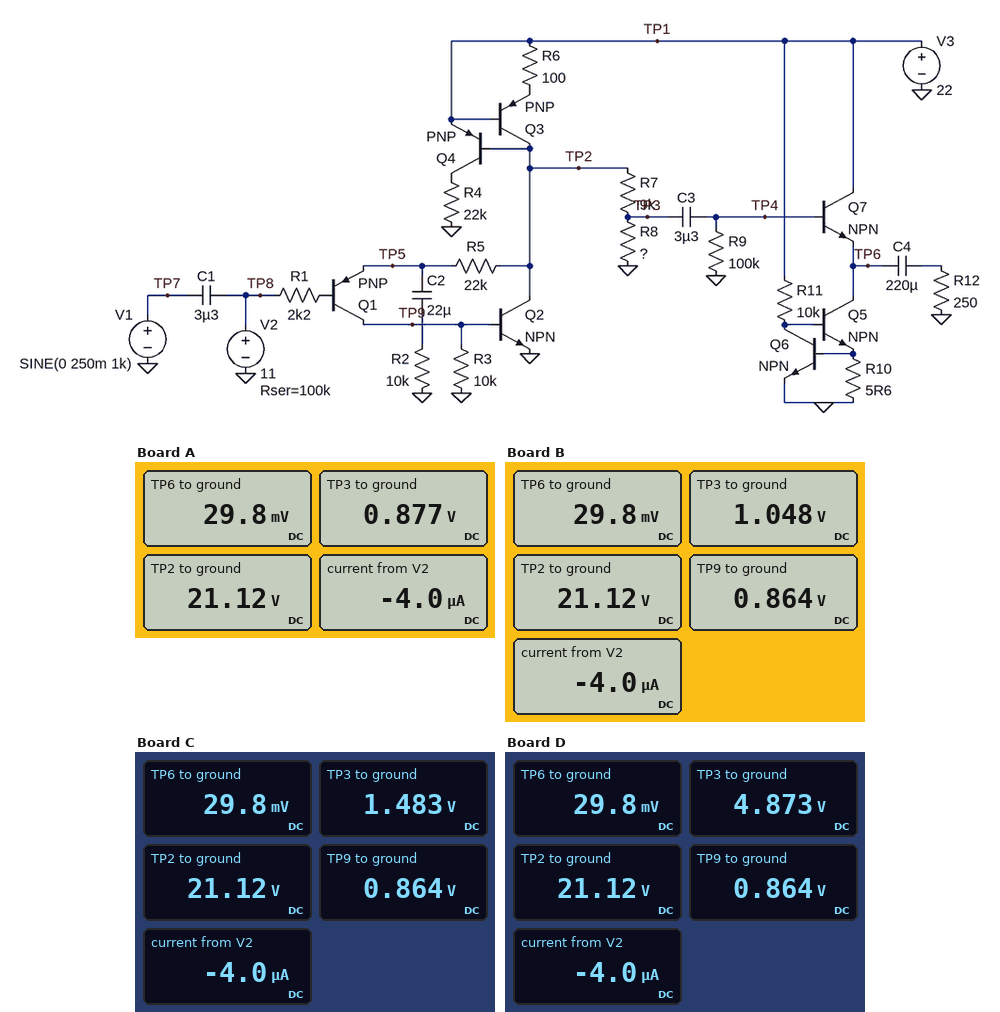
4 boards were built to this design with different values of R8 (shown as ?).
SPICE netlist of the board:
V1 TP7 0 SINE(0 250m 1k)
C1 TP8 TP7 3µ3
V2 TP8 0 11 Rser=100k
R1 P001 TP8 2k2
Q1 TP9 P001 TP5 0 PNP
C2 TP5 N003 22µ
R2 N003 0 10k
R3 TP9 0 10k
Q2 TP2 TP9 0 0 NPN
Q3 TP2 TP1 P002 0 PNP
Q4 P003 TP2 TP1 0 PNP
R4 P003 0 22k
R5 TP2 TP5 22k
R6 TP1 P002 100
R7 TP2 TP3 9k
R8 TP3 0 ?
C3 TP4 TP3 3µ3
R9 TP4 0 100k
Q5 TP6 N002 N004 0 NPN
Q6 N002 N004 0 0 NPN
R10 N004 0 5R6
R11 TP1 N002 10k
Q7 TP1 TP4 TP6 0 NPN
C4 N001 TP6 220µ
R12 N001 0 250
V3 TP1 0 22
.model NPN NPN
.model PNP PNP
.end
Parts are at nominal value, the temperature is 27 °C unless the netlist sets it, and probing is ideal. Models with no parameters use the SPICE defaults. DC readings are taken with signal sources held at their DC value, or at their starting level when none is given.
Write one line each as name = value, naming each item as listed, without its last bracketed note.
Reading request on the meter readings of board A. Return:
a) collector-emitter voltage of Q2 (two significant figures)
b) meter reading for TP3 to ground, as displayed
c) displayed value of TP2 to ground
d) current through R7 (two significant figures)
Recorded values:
collector-emitter voltage of Q2 = 21 V
meter reading for TP3 to ground, as displayed = 0.877 V
displayed value of TP2 to ground = 21.12 V
current through R7 = 2.2 mA
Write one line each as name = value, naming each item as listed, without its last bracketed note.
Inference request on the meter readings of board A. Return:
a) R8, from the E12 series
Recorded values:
R8, from the E12 series = 390 Ω
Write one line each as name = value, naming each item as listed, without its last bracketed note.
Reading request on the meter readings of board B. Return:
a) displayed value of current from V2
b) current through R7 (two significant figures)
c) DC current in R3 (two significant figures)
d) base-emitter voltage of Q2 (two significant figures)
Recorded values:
displayed value of current from V2 = -4.0 µA
current through R7 = 2.2 mA
DC current in R3 = 86 µA
base-emitter voltage of Q2 = 860 mV
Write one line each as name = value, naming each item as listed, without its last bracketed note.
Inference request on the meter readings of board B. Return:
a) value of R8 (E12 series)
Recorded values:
value of R8 = 470 Ω
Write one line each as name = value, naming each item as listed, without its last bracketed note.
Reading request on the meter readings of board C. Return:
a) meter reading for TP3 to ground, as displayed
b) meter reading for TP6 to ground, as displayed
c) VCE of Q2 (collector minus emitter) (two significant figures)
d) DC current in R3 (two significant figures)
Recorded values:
meter reading for TP3 to ground, as displayed = 1.483 V
meter reading for TP6 to ground, as displayed = 29.8 mV
VCE of Q2 (collector minus emitter) = 21 V
DC current in R3 = 86 µA
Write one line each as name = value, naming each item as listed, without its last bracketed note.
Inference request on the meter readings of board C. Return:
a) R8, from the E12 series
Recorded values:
R8, from the E12 series = 680 Ω
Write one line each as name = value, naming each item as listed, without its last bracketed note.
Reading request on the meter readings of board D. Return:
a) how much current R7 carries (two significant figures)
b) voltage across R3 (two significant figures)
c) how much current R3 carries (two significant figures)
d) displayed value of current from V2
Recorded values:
how much current R7 carries = 1.8 mA
voltage across R3 = 860 mV
how much current R3 carries = 86 µA
displayed value of current from V2 = -4.0 µA
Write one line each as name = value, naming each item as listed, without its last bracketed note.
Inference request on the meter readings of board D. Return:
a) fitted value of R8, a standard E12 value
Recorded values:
fitted value of R8, a standard E12 value = 2.7 kΩ
